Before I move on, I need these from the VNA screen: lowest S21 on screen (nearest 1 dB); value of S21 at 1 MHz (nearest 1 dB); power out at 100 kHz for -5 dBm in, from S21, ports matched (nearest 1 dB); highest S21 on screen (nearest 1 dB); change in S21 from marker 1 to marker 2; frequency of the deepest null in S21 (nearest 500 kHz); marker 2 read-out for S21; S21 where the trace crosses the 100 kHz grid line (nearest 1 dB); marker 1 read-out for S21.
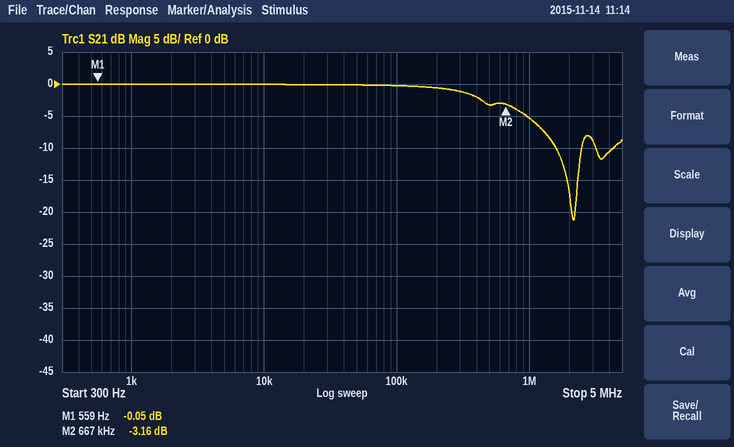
-21 dB
-5 dB
-5 dBm
0 dB
-3.11 dB
2.0 MHz
-3.16 dB
0 dB
-0.05 dB
